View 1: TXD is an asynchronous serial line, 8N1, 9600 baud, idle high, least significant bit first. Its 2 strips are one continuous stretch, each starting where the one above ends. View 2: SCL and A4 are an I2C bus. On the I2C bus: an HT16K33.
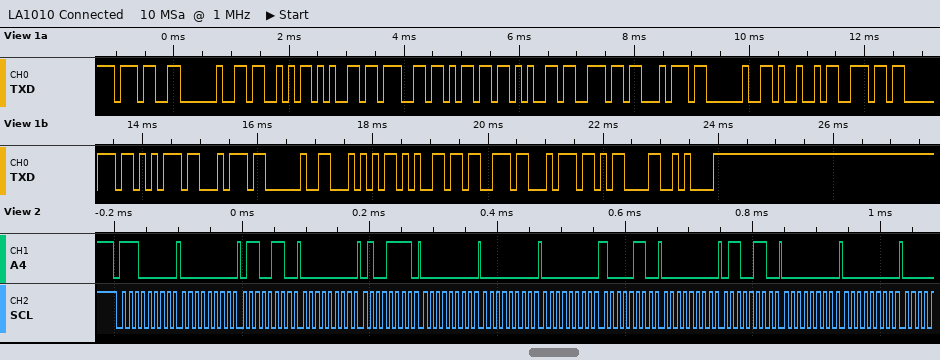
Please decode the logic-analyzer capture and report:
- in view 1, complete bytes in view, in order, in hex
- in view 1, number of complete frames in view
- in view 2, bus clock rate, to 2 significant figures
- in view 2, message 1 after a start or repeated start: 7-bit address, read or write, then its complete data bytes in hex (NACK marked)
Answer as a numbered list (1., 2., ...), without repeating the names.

1. 37 20 53 65 67 6D 65 6E 74 20 49 6E 70 75 74 20 54 65 73 74 0D 0A
2. 22
3. 100 kHz
4. 0x70 write: 00 66 00 4F 00 00 00 86 00 66 00 00
